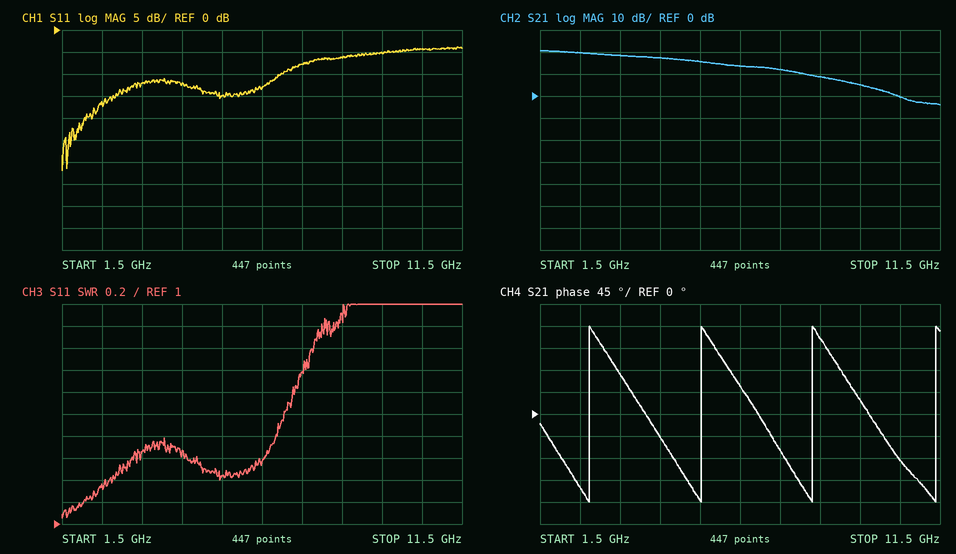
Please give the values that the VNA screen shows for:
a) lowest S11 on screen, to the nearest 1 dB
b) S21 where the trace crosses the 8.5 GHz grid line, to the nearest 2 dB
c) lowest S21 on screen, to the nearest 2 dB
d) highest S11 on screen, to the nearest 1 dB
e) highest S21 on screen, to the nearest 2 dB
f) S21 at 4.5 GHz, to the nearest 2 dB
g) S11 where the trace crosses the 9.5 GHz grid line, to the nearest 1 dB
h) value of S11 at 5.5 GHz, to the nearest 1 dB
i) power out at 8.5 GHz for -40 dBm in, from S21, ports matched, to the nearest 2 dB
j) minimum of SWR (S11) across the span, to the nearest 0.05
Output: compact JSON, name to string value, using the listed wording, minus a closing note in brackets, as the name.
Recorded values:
{"lowest S11 on screen, to the nearest 1 dB": "-32 dB", "S21 where the trace crosses the 8.5 GHz grid line, to the nearest 2 dB": "8 dB", "lowest S21 on screen, to the nearest 2 dB": "-4 dB", "highest S11 on screen, to the nearest 1 dB": "-4 dB", "highest S21 on screen, to the nearest 2 dB": "20 dB", "S21 at 4.5 GHz, to the nearest 2 dB": "18 dB", "S11 where the trace crosses the 9.5 GHz grid line, to the nearest 1 dB": "-5 dB", "value of S11 at 5.5 GHz, to the nearest 1 dB": "-15 dB", "power out at 8.5 GHz for -40 dBm in, from S21, ports matched, to the nearest 2 dB": "-32 dBm", "minimum of SWR (S11) across the span, to the nearest 0.05": "1.05"}
